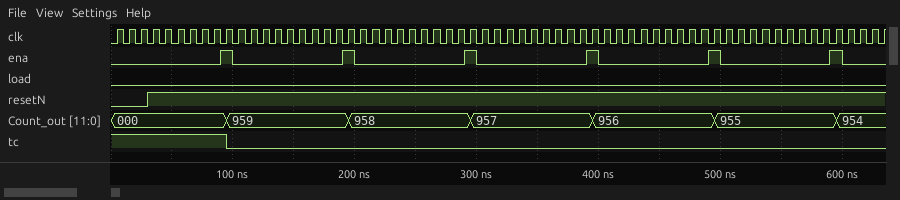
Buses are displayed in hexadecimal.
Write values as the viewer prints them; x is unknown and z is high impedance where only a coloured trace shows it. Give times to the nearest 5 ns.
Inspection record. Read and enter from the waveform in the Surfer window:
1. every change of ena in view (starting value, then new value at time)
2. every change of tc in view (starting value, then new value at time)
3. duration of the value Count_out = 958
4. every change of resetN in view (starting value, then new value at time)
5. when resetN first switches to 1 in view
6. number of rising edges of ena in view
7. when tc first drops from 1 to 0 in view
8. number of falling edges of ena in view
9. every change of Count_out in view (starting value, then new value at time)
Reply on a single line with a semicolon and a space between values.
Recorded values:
0, 1 at 90 ns, 0 at 100 ns, 1 at 190 ns, 0 at 200 ns, 1 at 290 ns, 0 at 300 ns, 1 at 390 ns, 0 at 400 ns, 1 at 490 ns, 0 at 500 ns, 1 at 590 ns, 0 at 600 ns; 1, 0 at 95 ns; 100 ns; 0, 1 at 30 ns; 30 ns; 6; 95 ns; 6; 000, 959 at 95 ns, 958 at 195 ns, 957 at 295 ns, 956 at 395 ns, 955 at 495 ns, 954 at 595 ns
